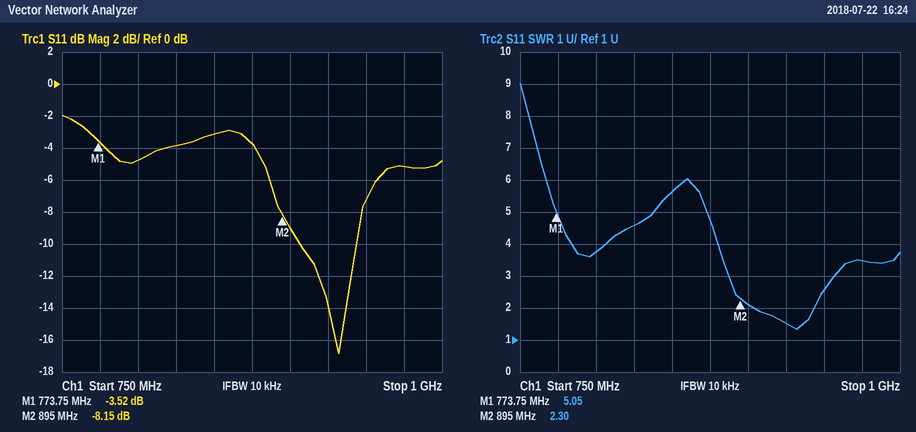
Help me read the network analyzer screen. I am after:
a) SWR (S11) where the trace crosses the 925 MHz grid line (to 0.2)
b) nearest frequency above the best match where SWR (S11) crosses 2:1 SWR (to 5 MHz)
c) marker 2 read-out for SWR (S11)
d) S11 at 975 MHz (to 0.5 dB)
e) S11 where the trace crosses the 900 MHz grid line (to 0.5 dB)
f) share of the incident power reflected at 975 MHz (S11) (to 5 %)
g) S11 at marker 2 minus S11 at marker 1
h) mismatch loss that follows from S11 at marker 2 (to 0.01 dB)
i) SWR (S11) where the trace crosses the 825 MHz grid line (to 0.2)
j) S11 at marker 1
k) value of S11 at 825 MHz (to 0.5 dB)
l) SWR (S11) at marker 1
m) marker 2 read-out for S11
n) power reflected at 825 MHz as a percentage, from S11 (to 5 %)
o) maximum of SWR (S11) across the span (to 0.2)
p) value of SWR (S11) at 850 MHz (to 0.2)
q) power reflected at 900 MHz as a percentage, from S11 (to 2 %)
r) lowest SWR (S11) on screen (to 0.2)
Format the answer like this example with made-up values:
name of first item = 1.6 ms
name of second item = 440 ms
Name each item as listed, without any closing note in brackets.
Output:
SWR (S11) where the trace crosses the 925 MHz grid line = 1.6
nearest frequency above the best match where SWR (S11) crosses 2:1 SWR = 945 MHz
marker 2 read-out for SWR = 2.30
S11 at 975 MHz = -5.0 dB
S11 where the trace crosses the 900 MHz grid line = -9.0 dB
share of the incident power reflected at 975 MHz (S11) = 30 %
S11 at marker 2 minus S11 at marker 1 = -4.63 dB
mismatch loss that follows from S11 at marker 2 = 0.72 dB
SWR (S11) where the trace crosses the 825 MHz grid line = 4.6
S11 at marker 1 = -3.52 dB
value of S11 at 825 MHz = -4.0 dB
SWR (S11) at marker 1 = 5.05
marker 2 read-out for S11 = -8.15 dB
power reflected at 825 MHz as a percentage, from S11 = 40 %
maximum of SWR (S11) across the span = 9.0
value of SWR (S11) at 850 MHz = 5.6
power reflected at 900 MHz as a percentage, from S11 = 12 %
lowest SWR (S11) on screen = 1.4
